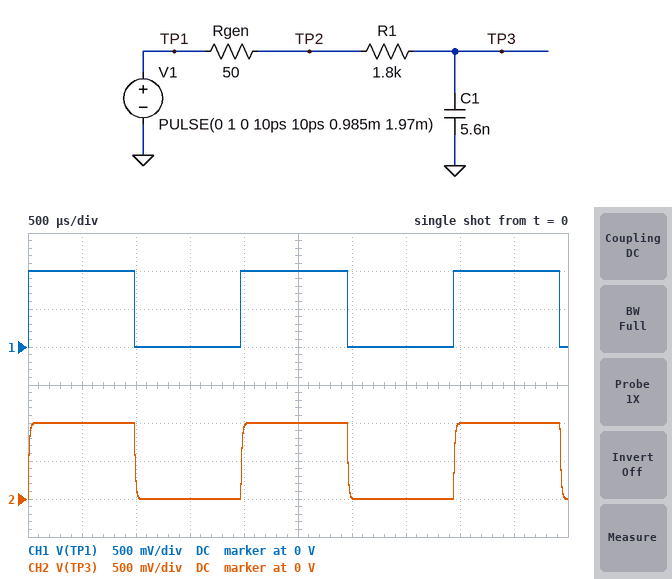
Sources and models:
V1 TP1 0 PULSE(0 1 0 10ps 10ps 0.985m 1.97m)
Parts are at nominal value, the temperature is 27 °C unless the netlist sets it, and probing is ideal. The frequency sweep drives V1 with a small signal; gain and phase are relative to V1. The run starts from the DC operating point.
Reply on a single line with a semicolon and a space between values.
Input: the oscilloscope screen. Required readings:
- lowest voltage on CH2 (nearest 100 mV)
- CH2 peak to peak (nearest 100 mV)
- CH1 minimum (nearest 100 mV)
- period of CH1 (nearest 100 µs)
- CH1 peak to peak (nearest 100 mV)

0 V; 1.0 V; 0 V; 2.0 ms; 1.0 V
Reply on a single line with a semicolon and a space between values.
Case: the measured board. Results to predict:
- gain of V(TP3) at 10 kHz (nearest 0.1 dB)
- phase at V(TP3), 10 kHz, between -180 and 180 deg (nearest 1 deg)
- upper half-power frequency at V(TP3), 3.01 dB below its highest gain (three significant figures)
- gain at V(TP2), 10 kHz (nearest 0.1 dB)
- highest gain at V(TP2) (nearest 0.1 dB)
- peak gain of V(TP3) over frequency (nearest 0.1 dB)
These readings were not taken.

-1.5 dB; -33 deg; 15.4 kHz; -0.1 dB; 0 dB; 0 dB
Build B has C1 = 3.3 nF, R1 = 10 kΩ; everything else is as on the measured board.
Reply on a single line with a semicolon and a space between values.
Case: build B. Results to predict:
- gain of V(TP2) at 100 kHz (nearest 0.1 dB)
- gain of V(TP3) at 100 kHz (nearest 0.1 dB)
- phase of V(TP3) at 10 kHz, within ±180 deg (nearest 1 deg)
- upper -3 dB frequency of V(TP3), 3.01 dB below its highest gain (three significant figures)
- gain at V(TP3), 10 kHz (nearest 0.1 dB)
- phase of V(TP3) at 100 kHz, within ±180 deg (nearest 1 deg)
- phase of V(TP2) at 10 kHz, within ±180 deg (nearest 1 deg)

0 dB; -26.4 dB; -64 deg; 4.80 kHz; -7.3 dB; -87 deg; 0 deg
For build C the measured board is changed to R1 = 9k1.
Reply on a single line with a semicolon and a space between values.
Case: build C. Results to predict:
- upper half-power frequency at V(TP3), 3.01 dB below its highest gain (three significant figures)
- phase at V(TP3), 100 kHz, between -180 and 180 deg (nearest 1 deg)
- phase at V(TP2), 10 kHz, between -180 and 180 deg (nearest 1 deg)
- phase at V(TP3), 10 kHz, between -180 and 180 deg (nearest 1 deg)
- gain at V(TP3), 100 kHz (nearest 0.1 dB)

3.11 kHz; -88 deg; 0 deg; -73 deg; -30.2 dB
